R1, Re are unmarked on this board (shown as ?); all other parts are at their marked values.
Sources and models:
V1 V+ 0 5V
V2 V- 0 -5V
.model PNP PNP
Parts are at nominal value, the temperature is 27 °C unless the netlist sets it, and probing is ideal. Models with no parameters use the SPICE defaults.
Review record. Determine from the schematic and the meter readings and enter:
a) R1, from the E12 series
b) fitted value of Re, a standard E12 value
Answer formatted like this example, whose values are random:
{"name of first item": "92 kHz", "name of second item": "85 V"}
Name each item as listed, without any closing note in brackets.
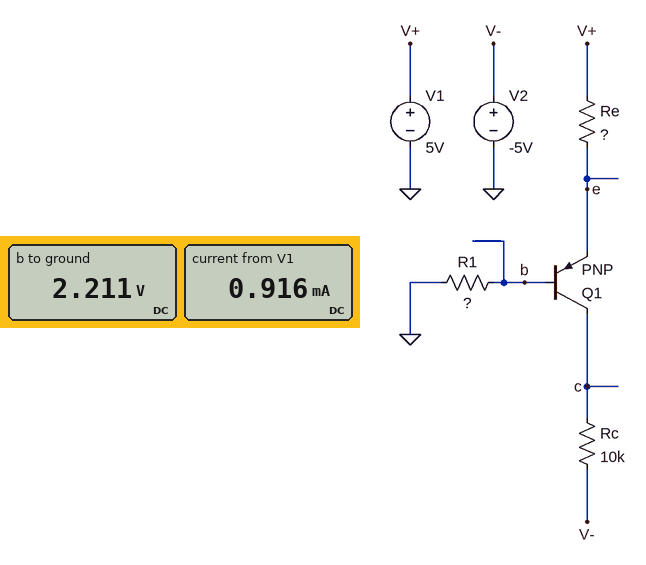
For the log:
{"R1, from the E12 series": "18 kΩ", "fitted value of Re, a standard E12 value": "2.2 kΩ"}
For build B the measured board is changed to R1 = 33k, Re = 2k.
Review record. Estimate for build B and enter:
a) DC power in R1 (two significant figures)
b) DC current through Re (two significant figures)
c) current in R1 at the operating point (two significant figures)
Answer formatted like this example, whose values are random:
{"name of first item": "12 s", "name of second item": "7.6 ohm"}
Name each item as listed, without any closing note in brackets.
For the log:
{"DC power in R1": "180 µW", "DC current through Re": "890 µA", "current in R1 at the operating point": "74 µA"}
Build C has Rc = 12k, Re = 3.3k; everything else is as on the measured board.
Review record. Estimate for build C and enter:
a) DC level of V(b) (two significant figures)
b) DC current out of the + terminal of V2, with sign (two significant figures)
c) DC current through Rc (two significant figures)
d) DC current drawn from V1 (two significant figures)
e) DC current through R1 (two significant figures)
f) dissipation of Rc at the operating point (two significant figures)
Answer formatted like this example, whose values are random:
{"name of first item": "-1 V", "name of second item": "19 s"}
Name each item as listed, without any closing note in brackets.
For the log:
{"DC level of V(b)": "1.8 V", "DC current out of the + terminal of V2, with sign": "-630 µA", "DC current through Rc": "630 µA", "DC current drawn from V1": "730 µA", "DC current through R1": "100 µA", "dissipation of Rc at the operating point": "4.7 mW"}
